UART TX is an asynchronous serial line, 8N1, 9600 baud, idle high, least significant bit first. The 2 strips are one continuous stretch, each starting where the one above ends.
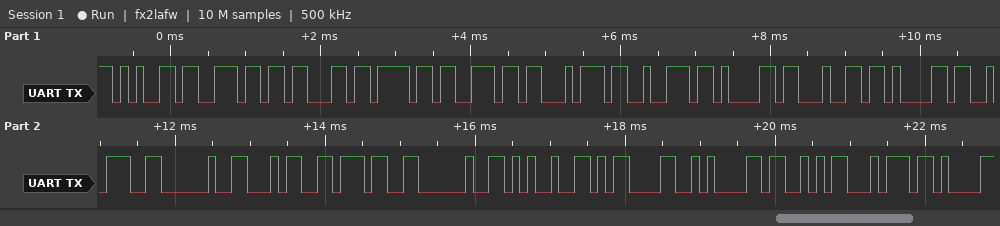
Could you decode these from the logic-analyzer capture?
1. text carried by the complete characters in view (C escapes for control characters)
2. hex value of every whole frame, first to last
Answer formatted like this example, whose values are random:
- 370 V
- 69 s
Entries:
- "encontrada: 47 %\r\nSt"
- 65 6E 63 6F 6E 74 72 61 64 61 3A 20 34 37 20 25 0D 0A 53 74
